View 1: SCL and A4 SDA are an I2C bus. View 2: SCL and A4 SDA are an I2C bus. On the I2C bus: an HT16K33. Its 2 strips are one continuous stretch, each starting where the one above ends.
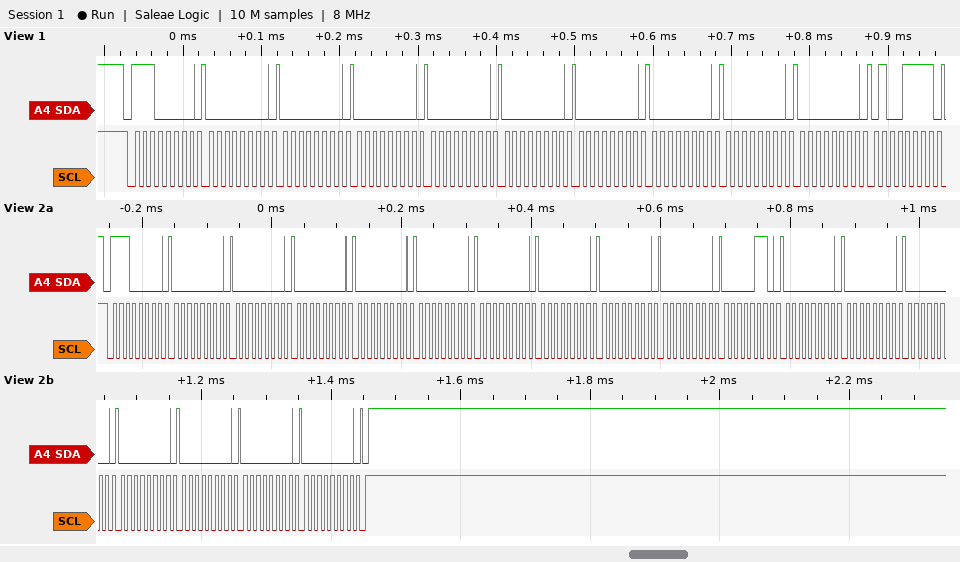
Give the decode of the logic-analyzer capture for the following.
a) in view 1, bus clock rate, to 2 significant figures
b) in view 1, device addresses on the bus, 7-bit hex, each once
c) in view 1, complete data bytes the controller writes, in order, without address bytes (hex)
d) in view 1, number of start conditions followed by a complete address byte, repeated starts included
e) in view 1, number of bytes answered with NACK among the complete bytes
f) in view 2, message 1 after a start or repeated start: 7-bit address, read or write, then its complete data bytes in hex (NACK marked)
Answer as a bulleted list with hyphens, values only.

- 100 kHz
- 0x70
- 00 00 00 00 00 00 00 00 00 4F
- 1
- 0
- 0x70 write: 00 00 00 00 00 00 00 00 00 06 00 00 00 00 00 00 00
